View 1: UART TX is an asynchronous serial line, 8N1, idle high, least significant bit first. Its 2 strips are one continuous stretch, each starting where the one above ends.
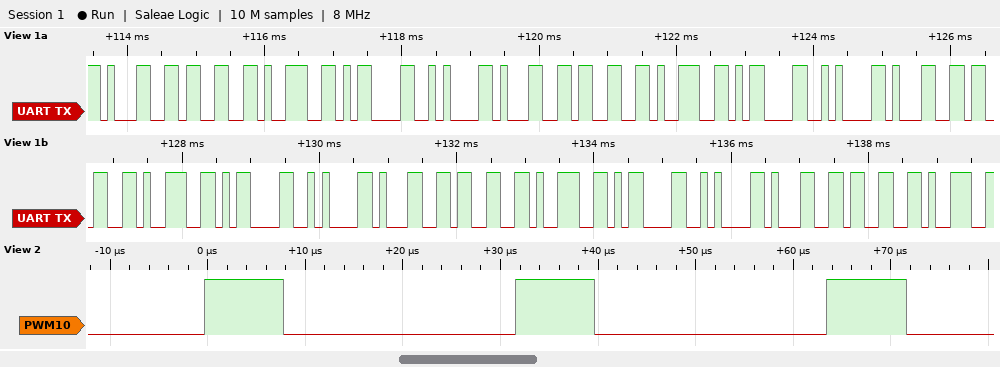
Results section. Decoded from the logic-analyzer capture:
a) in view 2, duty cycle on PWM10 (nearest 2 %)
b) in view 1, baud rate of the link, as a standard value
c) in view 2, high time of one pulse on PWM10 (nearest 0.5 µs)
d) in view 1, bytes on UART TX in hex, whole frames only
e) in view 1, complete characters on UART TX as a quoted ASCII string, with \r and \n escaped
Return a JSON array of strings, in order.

["26 %", "9600 baud", "8.0 µs", "31 33 39 0D 0A 31 33 39 0D 0A 31 33 39 0D 0A 31 33 39 0D 0A 31 33 39", "\"139\\r\\n139\\r\\n139\\r\\n139\\r\\n139\""]
